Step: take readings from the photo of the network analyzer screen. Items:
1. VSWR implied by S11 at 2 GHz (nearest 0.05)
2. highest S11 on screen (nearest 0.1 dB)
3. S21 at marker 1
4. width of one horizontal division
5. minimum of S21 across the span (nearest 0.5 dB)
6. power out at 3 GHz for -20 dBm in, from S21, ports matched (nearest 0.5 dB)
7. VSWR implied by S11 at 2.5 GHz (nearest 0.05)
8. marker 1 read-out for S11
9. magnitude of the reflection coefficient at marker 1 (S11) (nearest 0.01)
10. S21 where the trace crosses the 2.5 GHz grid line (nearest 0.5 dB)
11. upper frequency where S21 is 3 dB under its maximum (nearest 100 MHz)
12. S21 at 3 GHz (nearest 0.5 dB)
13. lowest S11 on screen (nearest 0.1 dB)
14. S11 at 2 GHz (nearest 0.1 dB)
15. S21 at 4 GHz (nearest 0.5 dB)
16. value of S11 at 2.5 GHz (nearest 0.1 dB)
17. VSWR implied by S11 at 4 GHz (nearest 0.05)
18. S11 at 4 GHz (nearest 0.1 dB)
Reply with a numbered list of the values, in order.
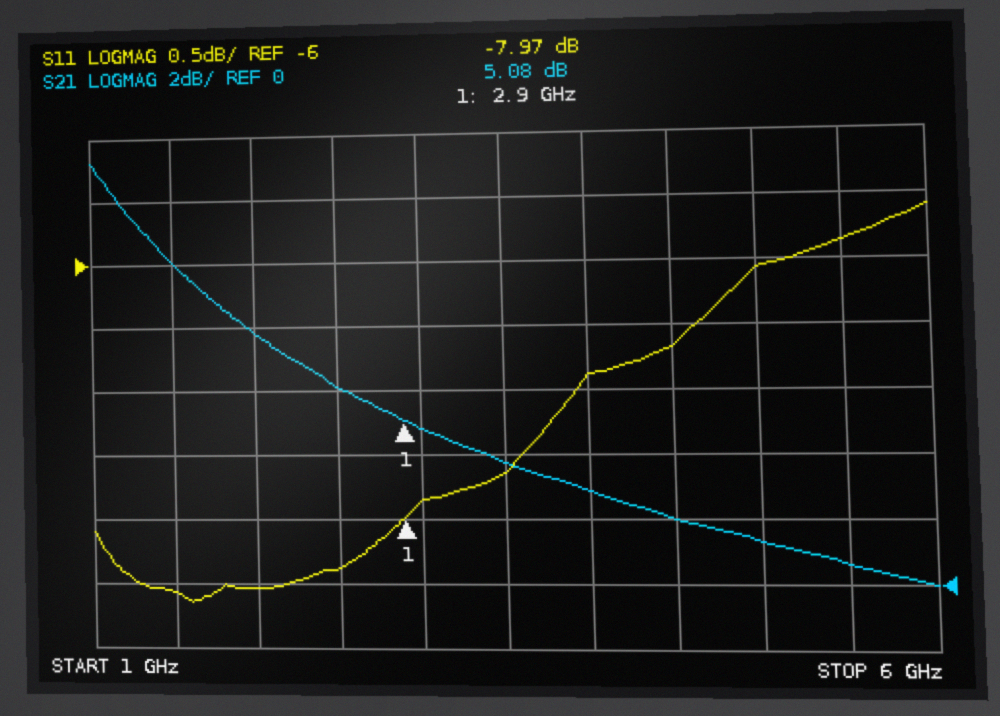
1. 2.20
2. -5.6 dB
3. 5.08 dB
4. 500 MHz
5. 0.0 dB
6. -15.0 dBm
7. 2.25
8. -7.97 dB
9. 0.40
10. 6.0 dB
11. 1.5 GHz
12. 5.0 dB
13. -8.6 dB
14. -8.5 dB
15. 3.0 dB
16. -8.4 dB
17. 2.65
18. -6.9 dB
